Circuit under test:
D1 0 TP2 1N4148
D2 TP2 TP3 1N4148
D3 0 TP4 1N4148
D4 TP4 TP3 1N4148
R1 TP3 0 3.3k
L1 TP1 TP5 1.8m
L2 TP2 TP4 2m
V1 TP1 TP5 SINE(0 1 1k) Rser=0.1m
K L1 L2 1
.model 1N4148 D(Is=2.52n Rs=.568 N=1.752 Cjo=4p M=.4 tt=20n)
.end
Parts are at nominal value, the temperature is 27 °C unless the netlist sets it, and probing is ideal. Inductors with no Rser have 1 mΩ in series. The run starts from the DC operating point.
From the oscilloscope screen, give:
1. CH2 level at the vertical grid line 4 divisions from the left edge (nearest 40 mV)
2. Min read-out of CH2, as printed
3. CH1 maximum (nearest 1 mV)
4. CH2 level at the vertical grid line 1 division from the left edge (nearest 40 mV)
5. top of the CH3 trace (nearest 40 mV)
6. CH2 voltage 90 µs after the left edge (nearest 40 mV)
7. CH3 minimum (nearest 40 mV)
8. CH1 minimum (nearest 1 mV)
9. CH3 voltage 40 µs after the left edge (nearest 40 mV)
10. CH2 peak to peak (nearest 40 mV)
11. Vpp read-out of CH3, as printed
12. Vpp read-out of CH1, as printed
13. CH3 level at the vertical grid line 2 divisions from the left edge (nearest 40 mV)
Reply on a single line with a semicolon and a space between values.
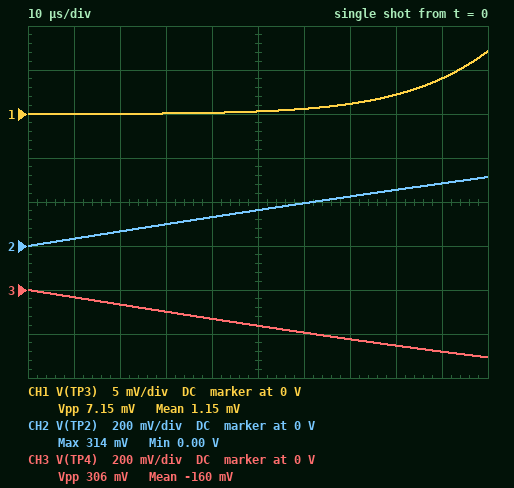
120 mV; 0.00 V; 7 mV; 40 mV; 0 V; 280 mV; -320 mV; 0 V; -120 mV; 320 mV; 306 mV; 7.15 mV; -80 mV
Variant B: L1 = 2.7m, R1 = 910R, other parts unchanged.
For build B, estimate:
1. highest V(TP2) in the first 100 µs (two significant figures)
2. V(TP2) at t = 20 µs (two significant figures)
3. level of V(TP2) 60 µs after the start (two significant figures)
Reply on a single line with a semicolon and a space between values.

250 mV; 54 mV; 160 mV
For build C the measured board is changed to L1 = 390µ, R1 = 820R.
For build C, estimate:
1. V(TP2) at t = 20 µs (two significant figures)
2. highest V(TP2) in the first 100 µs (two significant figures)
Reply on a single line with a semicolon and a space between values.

140 mV; 800 mV
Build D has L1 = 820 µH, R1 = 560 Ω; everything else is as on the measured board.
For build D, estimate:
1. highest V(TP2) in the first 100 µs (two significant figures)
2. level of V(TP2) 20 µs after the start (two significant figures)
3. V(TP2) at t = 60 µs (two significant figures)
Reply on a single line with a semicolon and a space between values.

470 mV; 98 mV; 290 mV
